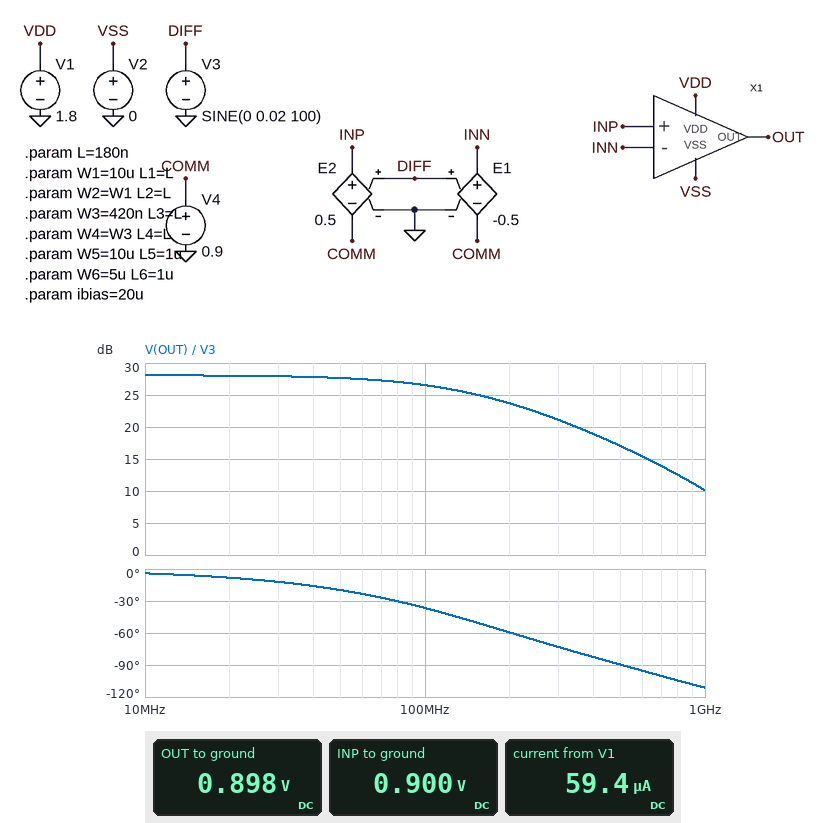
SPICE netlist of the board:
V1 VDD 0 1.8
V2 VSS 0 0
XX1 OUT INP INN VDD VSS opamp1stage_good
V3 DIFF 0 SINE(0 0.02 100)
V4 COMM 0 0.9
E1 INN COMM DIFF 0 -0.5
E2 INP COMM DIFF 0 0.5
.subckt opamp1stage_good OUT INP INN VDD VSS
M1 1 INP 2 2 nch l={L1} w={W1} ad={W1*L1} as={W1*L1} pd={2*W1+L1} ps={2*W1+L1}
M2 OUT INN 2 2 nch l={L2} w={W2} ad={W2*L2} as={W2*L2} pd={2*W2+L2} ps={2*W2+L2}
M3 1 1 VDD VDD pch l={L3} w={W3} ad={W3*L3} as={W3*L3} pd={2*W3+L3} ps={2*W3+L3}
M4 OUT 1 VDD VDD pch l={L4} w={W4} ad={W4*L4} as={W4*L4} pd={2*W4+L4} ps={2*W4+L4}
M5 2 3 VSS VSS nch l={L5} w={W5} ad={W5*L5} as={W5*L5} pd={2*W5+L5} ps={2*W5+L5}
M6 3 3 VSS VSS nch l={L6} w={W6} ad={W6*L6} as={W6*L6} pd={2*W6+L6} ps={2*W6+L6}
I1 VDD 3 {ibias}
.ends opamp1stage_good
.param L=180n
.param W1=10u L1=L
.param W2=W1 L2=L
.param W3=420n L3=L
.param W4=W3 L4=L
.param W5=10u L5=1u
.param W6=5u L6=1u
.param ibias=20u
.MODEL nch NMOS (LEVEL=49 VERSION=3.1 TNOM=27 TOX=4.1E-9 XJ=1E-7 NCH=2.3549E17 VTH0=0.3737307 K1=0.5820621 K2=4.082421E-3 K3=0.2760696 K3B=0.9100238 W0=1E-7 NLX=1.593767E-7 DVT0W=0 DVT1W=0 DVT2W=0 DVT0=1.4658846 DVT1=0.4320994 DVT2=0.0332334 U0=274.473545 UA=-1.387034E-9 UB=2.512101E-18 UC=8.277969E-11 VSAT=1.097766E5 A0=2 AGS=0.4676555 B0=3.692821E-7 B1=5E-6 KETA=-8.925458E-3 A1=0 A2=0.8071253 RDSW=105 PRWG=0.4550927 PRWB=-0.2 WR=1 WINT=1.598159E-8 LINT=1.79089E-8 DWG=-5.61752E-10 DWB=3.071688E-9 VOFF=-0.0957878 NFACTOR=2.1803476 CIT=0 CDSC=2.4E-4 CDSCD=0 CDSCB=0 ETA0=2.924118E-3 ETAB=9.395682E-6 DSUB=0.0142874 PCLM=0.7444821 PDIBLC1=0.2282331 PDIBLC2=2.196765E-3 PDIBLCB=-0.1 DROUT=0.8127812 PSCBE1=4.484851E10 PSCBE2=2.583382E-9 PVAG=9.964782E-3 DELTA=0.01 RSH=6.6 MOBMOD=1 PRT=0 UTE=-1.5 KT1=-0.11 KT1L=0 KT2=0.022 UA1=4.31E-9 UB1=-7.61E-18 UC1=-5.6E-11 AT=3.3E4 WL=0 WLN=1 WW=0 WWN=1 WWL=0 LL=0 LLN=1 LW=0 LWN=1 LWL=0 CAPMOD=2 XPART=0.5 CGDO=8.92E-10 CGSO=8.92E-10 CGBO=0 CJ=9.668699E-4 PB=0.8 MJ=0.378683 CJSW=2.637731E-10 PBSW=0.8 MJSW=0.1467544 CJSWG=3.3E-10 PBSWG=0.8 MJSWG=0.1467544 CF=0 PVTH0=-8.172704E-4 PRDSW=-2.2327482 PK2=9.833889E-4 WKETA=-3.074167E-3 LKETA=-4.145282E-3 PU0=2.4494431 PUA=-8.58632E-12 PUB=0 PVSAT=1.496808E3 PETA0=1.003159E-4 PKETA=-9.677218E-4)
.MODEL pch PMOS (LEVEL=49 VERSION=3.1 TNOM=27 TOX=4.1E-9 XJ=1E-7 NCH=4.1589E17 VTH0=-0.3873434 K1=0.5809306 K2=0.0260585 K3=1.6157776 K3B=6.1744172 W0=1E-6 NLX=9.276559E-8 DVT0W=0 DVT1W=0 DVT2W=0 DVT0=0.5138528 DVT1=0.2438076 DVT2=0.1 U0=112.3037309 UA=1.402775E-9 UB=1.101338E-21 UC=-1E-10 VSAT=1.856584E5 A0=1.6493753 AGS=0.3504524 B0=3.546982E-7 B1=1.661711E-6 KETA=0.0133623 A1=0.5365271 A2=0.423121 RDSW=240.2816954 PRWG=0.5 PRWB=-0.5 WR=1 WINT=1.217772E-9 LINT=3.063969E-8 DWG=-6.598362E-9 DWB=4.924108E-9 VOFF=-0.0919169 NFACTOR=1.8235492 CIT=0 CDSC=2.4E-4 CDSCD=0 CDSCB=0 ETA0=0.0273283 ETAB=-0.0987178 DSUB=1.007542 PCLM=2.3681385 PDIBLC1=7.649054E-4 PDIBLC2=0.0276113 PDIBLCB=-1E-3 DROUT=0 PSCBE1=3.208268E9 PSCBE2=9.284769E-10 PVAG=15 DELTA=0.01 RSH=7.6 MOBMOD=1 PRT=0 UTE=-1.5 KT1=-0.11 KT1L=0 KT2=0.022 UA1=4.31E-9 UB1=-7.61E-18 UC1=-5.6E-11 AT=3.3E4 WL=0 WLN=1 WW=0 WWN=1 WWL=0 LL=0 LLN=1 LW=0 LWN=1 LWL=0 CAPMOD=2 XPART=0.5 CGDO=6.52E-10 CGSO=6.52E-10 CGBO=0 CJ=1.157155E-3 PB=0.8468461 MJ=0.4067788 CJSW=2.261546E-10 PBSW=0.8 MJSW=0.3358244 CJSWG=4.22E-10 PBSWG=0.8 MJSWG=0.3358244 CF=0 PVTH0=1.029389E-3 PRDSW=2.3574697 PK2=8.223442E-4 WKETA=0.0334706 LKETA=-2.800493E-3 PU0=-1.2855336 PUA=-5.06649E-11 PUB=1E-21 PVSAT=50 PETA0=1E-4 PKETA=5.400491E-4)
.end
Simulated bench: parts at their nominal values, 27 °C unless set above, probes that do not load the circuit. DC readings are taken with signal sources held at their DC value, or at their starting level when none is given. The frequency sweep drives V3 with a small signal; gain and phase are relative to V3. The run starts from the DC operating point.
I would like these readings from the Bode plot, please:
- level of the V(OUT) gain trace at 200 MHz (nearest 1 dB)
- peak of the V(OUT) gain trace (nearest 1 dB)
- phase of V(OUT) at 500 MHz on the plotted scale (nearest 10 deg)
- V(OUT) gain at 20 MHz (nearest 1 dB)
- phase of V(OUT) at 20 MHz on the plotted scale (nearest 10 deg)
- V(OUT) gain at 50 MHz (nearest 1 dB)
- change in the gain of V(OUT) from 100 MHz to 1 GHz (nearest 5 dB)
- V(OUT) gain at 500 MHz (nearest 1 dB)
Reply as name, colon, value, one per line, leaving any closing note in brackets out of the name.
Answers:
level of the V(OUT) gain trace at 200 MHz: 24 dB
peak of the V(OUT) gain trace: 28 dB
phase of V(OUT) at 500 MHz on the plotted scale: -90 deg
V(OUT) gain at 20 MHz: 28 dB
phase of V(OUT) at 20 MHz on the plotted scale: -10 deg
V(OUT) gain at 50 MHz: 28 dB
change in the gain of V(OUT) from 100 MHz to 1 GHz: -15 dB
V(OUT) gain at 500 MHz: 17 dB
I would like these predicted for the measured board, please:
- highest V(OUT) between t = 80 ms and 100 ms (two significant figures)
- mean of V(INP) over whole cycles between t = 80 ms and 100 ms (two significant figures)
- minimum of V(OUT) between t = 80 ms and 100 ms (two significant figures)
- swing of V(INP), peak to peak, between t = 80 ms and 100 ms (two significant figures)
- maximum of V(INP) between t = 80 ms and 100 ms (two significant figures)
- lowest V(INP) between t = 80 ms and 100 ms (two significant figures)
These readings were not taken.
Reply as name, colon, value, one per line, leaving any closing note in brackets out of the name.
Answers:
highest V(OUT) between t = 80 ms and 100 ms: 1.4 V
mean of V(INP) over whole cycles between t = 80 ms and 100 ms: 900 mV
minimum of V(OUT) between t = 80 ms and 100 ms: 490 mV
swing of V(INP), peak to peak, between t = 80 ms and 100 ms: 20 mV
maximum of V(INP) between t = 80 ms and 100 ms: 910 mV
lowest V(INP) between t = 80 ms and 100 ms: 890 mV
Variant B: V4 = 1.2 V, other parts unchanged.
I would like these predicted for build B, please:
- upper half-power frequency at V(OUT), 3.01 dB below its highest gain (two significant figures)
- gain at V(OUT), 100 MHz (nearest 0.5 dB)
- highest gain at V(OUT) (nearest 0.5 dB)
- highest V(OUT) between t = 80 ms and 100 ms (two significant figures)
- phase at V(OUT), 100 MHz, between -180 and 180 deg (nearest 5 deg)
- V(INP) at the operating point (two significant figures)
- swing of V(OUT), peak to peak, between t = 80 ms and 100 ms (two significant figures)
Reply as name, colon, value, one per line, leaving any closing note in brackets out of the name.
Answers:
upper half-power frequency at V(OUT), 3.01 dB below its highest gain: 190 MHz
gain at V(OUT), 100 MHz: 25.0 dB
highest gain at V(OUT): 26.0 dB
highest V(OUT) between t = 80 ms and 100 ms: 1.3 V
phase at V(OUT), 100 MHz, between -180 and 180 deg: -30 deg
V(INP) at the operating point: 1.2 V
swing of V(OUT), peak to peak, between t = 80 ms and 100 ms: 590 mV
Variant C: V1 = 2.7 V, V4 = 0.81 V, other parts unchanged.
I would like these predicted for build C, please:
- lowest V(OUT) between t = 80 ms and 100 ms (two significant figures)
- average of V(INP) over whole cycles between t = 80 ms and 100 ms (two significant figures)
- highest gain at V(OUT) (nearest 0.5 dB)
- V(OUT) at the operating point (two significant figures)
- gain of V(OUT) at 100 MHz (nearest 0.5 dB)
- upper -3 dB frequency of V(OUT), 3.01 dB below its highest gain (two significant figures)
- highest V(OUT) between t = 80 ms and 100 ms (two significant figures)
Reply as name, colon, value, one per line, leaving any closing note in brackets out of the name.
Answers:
lowest V(OUT) between t = 80 ms and 100 ms: 1.2 V
average of V(INP) over whole cycles between t = 80 ms and 100 ms: 810 mV
highest gain at V(OUT): 30.0 dB
V(OUT) at the operating point: 1.8 V
gain of V(OUT) at 100 MHz: 28.0 dB
upper -3 dB frequency of V(OUT), 3.01 dB below its highest gain: 130 MHz
highest V(OUT) between t = 80 ms and 100 ms: 2.3 V
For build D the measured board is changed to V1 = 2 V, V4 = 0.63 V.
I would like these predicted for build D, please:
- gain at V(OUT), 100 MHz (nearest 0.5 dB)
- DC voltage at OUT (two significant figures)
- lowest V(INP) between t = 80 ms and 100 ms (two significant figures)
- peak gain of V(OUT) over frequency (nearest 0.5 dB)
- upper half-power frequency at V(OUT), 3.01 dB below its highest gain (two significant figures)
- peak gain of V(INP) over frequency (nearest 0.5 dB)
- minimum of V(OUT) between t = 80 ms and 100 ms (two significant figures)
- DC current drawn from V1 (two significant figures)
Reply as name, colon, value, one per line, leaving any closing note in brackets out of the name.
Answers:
gain at V(OUT), 100 MHz: 27.0 dB
DC voltage at OUT: 1.1 V
lowest V(INP) between t = 80 ms and 100 ms: 620 mV
peak gain of V(OUT) over frequency: 29.0 dB
upper half-power frequency at V(OUT), 3.01 dB below its highest gain: 130 MHz
peak gain of V(INP) over frequency: -6.0 dB
minimum of V(OUT) between t = 80 ms and 100 ms: 560 mV
DC current drawn from V1: 57 µA
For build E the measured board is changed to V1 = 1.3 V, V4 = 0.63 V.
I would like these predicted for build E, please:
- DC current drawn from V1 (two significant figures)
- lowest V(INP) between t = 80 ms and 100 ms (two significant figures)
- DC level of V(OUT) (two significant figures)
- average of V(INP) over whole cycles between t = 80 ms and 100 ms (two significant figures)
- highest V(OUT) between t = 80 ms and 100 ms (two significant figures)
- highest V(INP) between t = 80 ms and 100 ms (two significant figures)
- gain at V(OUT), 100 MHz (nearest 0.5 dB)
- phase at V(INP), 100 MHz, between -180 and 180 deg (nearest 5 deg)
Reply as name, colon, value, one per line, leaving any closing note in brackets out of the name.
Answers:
DC current drawn from V1: 56 µA
lowest V(INP) between t = 80 ms and 100 ms: 620 mV
DC level of V(OUT): 420 mV
average of V(INP) over whole cycles between t = 80 ms and 100 ms: 630 mV
highest V(OUT) between t = 80 ms and 100 ms: 870 mV
highest V(INP) between t = 80 ms and 100 ms: 640 mV
gain at V(OUT), 100 MHz: 25.5 dB
phase at V(INP), 100 MHz, between -180 and 180 deg: 0 deg
